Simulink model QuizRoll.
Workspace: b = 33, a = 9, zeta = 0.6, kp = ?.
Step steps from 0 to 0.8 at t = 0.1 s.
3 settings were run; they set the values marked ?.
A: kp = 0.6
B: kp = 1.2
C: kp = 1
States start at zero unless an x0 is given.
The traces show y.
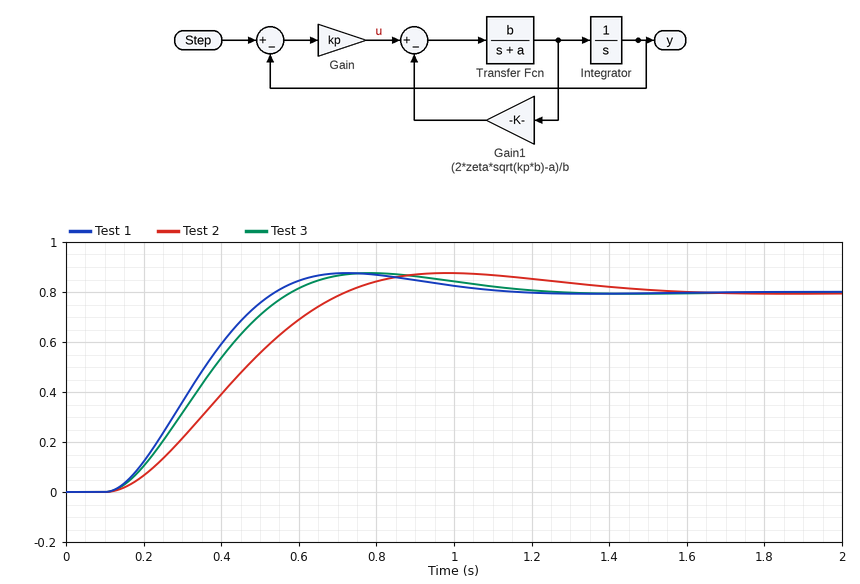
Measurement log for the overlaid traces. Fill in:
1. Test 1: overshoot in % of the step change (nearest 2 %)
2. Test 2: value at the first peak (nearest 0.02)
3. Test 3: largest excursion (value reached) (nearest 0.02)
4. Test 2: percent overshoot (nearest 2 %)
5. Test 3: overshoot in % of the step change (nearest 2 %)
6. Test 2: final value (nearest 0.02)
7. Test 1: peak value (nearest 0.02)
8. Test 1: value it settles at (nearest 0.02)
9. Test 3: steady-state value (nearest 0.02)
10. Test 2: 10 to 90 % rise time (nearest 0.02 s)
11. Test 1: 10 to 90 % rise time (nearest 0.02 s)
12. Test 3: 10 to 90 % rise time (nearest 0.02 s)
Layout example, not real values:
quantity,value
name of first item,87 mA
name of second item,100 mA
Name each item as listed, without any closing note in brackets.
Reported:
quantity,value
Test 1: overshoot in % of the step change,10 %
Test 2: value at the first peak,0.88
Test 3: largest excursion (value reached),0.88
Test 2: percent overshoot,10 %
Test 3: overshoot in % of the step change,10 %
Test 2: final value,0.80
Test 1: peak value,0.88
Test 1: value it settles at,0.80
Test 3: steady-state value,0.80
Test 2: 10 to 90 % rise time,0.42 s
Test 1: 10 to 90 % rise time,0.30 s
Test 3: 10 to 90 % rise time,0.32 s
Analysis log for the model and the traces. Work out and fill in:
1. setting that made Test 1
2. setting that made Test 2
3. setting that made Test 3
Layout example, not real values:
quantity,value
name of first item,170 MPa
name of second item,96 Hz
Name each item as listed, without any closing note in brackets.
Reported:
quantity,value
setting that made Test 1,B
setting that made Test 2,A
setting that made Test 3,C
